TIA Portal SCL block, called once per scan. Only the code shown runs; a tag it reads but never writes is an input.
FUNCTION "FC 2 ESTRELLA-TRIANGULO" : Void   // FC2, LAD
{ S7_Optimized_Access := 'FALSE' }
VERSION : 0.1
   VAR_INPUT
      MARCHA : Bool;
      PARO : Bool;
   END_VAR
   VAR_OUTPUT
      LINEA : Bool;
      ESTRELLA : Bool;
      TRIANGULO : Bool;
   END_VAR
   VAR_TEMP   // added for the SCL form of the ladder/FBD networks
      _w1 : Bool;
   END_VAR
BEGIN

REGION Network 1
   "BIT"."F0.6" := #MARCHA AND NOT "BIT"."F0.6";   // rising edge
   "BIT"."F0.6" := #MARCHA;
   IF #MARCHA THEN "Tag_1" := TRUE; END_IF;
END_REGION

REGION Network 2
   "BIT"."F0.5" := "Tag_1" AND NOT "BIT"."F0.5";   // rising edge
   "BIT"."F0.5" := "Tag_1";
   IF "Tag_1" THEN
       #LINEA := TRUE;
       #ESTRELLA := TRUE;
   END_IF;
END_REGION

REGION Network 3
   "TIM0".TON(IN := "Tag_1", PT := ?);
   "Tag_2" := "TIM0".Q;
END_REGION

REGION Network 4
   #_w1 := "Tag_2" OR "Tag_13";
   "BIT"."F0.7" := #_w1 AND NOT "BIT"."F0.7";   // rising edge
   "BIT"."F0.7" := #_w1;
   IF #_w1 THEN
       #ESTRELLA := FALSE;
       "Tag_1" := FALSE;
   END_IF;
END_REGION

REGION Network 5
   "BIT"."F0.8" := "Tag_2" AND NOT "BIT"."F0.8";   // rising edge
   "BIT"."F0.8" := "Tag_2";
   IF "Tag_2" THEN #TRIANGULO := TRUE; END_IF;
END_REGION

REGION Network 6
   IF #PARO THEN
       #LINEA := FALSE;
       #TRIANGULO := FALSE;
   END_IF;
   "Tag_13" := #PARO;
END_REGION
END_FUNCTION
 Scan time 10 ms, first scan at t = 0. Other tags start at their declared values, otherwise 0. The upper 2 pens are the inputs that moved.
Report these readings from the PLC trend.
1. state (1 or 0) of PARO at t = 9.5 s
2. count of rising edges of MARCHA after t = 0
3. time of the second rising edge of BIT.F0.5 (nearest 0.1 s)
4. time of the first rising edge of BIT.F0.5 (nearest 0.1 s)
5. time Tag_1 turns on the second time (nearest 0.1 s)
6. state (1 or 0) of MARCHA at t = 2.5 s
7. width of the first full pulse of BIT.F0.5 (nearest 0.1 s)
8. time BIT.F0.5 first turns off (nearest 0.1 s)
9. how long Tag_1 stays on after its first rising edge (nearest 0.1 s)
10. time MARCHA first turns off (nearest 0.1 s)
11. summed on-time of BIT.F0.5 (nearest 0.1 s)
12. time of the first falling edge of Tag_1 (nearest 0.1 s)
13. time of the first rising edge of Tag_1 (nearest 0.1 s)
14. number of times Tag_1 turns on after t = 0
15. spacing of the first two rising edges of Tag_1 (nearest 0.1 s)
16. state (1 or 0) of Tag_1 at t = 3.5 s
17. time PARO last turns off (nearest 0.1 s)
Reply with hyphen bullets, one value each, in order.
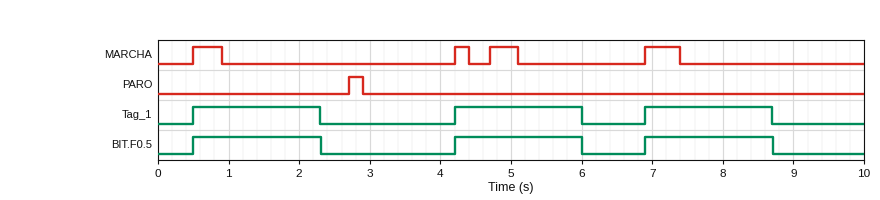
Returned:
- 0
- 4
- 4.2 s
- 0.5 s
- 4.2 s
- 0
- 1.8 s
- 2.3 s
- 1.8 s
- 0.9 s
- 5.4 s
- 2.3 s
- 0.5 s
- 3
- 3.7 s
- 0
- 2.9 s
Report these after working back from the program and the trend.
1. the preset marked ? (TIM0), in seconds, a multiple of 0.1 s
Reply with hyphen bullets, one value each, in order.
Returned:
- 1.8 s
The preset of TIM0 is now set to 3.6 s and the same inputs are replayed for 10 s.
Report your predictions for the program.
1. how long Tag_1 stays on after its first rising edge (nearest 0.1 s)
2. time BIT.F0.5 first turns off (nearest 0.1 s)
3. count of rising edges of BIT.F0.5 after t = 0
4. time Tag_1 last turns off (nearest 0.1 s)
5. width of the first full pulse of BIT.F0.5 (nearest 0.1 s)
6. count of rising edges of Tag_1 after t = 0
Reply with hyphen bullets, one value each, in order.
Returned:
- 2.2 s
- 2.7 s
- 2
- 7.8 s
- 2.2 s
- 2
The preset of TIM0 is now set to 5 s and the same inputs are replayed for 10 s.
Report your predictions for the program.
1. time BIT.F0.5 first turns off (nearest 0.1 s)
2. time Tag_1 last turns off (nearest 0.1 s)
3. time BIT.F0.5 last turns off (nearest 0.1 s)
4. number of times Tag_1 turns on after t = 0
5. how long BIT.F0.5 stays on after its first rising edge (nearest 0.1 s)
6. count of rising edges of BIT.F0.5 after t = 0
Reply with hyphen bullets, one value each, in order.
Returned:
- 2.7 s
- 9.2 s
- 9.2 s
- 2
- 2.2 s
- 2
